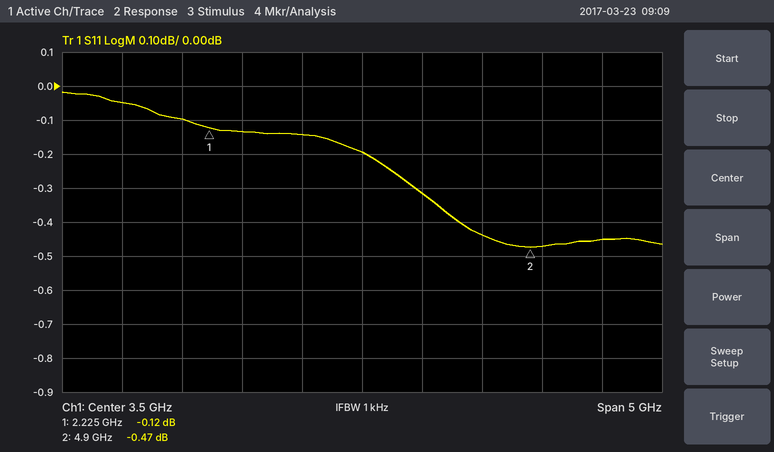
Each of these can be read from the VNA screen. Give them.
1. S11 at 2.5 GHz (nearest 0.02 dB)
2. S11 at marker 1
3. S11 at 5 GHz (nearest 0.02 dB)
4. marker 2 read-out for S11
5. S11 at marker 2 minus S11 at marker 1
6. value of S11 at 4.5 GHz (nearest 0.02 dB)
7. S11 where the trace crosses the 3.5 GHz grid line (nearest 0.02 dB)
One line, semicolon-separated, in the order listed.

-0.14 dB; -0.12 dB; -0.48 dB; -0.47 dB; -0.35 dB; -0.44 dB; -0.20 dB
